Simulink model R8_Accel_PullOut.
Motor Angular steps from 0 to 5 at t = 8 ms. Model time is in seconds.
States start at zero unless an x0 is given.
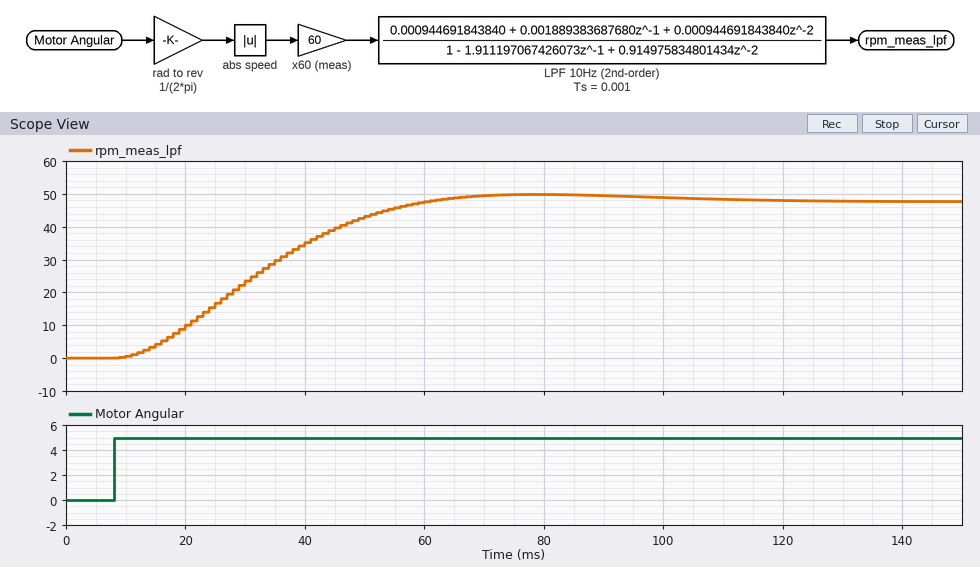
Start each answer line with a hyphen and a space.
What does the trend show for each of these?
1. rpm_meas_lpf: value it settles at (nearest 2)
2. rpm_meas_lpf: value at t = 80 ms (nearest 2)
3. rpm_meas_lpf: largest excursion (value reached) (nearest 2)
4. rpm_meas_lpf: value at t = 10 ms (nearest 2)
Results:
- 48
- 50
- 50
- 0
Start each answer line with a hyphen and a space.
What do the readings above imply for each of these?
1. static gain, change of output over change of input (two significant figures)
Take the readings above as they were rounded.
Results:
- 9.6
